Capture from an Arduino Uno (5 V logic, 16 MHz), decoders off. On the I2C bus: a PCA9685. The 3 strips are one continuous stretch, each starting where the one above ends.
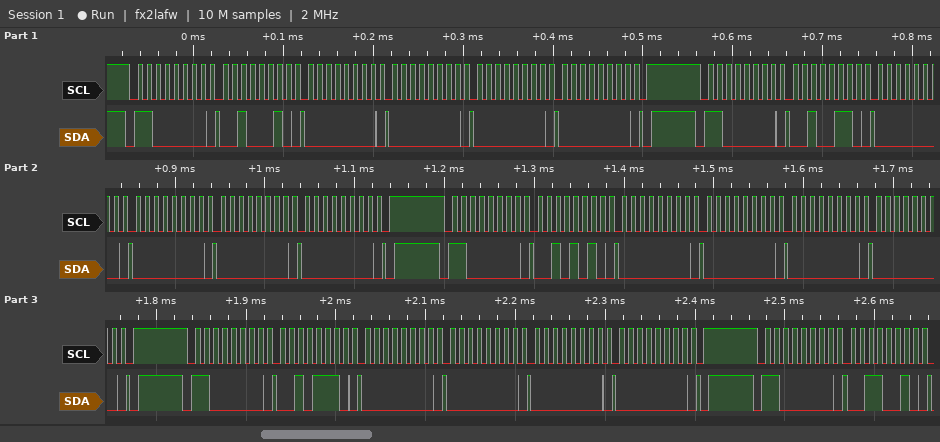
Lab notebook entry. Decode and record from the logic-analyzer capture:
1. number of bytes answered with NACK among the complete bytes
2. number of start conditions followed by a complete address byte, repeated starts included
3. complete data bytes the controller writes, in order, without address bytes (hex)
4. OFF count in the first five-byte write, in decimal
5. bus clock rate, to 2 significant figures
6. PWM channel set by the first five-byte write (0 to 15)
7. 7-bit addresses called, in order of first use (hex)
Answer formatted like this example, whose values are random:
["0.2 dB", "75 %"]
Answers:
["0", "5", "22 00 00 00 00 26 00 00 00 00 2A 00 00 00 00 2E 00 00 00 00 32", "0", "100 kHz", "7", "0x60"]
